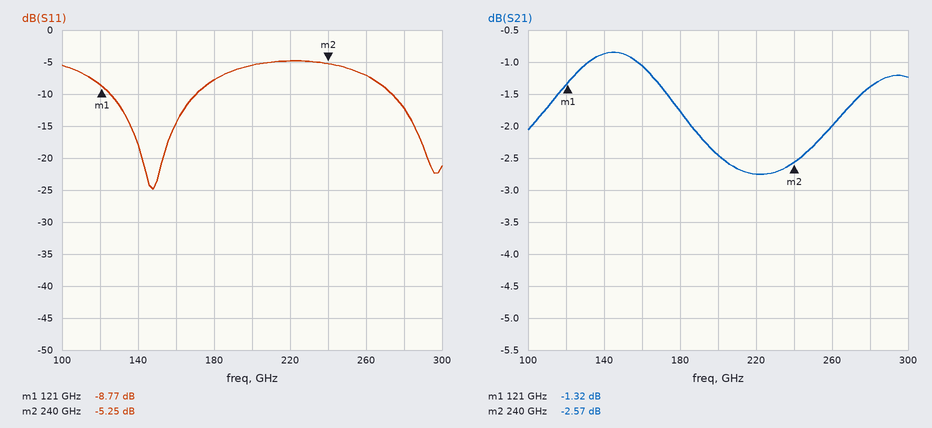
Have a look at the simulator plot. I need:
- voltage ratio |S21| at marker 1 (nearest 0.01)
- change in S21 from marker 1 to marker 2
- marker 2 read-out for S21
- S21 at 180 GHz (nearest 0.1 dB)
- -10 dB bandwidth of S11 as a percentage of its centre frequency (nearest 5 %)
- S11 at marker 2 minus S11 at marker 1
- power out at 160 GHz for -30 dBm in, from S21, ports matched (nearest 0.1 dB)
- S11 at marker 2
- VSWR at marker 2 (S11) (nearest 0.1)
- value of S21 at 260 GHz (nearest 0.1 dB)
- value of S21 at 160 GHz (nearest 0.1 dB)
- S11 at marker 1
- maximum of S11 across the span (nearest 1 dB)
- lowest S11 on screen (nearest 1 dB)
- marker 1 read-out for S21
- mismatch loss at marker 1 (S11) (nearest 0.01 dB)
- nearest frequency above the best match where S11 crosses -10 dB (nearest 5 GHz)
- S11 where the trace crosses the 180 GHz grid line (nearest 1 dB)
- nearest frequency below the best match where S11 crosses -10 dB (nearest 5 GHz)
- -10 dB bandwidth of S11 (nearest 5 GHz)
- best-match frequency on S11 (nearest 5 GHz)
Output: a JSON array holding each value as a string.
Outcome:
["0.86", "-1.25 dB", "-2.57 dB", "-1.8 dB", "30 %", "3.52 dB", "-31.1 dBm", "-5.25 dB", "3.4", "-2.0 dB", "-1.1 dB", "-8.77 dB", "-5 dB", "-25 dB", "-1.32 dB", "0.62 dB", "170 GHz", "-8 dB", "125 GHz", "45 GHz", "150 GHz"]
